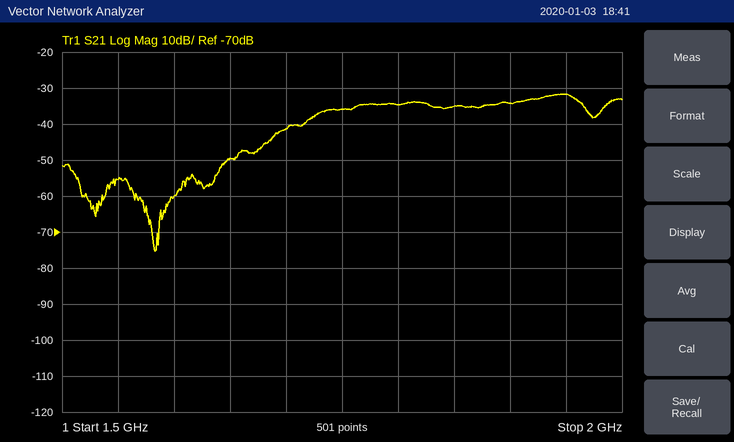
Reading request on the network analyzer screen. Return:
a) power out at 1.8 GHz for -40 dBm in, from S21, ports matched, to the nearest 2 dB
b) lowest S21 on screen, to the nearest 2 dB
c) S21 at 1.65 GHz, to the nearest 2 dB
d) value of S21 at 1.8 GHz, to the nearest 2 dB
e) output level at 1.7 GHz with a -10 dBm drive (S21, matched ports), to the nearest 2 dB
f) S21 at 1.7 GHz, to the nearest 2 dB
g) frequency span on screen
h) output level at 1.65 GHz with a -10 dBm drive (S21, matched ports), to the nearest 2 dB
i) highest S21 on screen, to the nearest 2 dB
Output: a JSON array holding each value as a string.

["-74 dBm", "-76 dB", "-50 dB", "-34 dB", "-52 dBm", "-42 dB", "500 MHz", "-60 dBm", "-32 dB"]
